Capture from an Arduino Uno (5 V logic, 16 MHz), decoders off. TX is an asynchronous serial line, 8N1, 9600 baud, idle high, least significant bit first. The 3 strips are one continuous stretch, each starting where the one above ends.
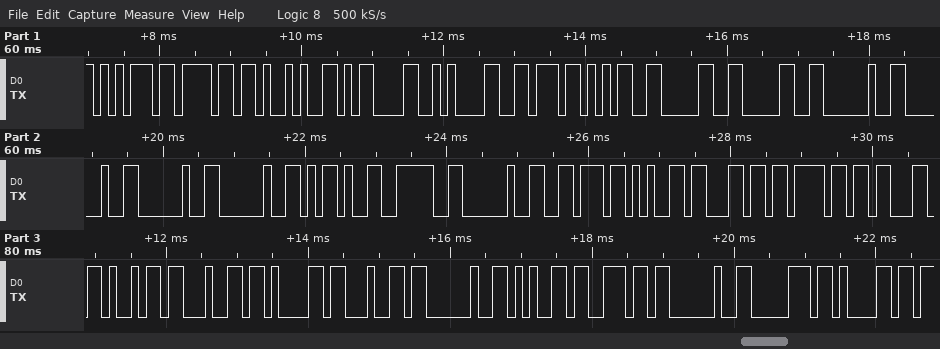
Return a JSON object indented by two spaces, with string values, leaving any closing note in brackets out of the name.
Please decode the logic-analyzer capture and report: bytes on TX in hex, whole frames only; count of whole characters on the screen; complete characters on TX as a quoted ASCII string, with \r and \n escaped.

{
  "bytes on TX in hex, whole frames only": "75 6F 29 0D 0A 76 35 30 30 20 20 20 20 2D 3E 20 76 65 6C 6F 63 69 64 61 64 20 65 6E 20 70 61",
  "count of whole characters on the screen": "31",
  "complete characters on TX as a quoted ASCII string, with \\r and \\n escaped": "\"uo)\\r\\nv500    -> velocidad en pa\""
}
